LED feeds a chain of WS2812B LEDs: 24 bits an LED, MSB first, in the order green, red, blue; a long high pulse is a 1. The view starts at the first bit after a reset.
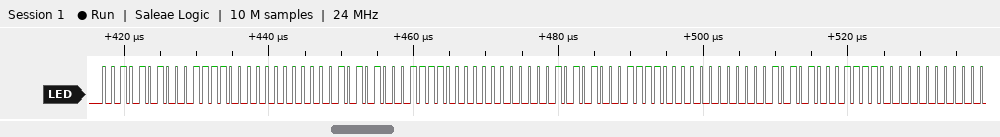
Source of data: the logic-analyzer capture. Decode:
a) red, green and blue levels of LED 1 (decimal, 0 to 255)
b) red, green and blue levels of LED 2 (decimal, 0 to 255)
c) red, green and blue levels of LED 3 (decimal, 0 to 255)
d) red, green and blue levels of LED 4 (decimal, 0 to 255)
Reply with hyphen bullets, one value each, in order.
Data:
- 60, 42, 0
- 60, 42, 0
- 60, 42, 0
- 60, 42, 0
